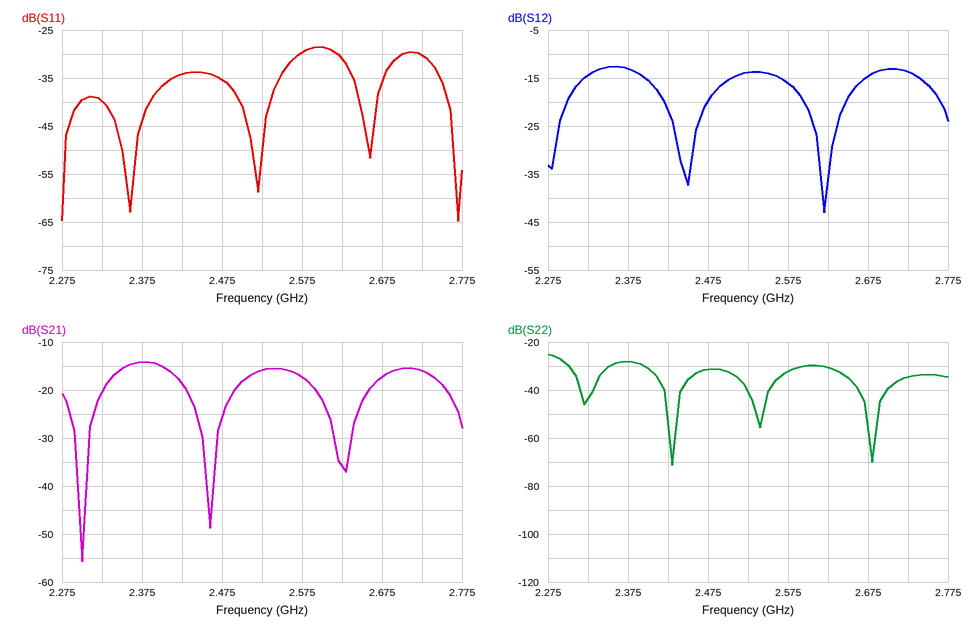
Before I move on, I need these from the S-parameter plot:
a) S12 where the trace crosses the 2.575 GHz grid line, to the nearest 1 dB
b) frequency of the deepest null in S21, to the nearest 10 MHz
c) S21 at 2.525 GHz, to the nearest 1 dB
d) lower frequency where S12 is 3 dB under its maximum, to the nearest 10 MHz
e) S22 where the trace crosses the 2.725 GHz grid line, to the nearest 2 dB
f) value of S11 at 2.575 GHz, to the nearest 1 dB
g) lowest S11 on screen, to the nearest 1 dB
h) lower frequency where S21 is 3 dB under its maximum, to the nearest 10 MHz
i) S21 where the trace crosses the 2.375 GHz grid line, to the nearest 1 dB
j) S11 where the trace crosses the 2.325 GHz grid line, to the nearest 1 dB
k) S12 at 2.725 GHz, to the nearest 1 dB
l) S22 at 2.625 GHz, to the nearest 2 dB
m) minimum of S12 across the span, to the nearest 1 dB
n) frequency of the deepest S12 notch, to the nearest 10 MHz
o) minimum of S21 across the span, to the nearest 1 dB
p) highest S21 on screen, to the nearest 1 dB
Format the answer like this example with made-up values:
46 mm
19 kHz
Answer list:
-16 dB
2.30 GHz
-16 dB
2.32 GHz
-34 dB
-30 dB
-65 dB
2.34 GHz
-14 dB
-40 dB
-14 dB
-30 dB
-43 dB
2.62 GHz
-56 dB
-14 dB
